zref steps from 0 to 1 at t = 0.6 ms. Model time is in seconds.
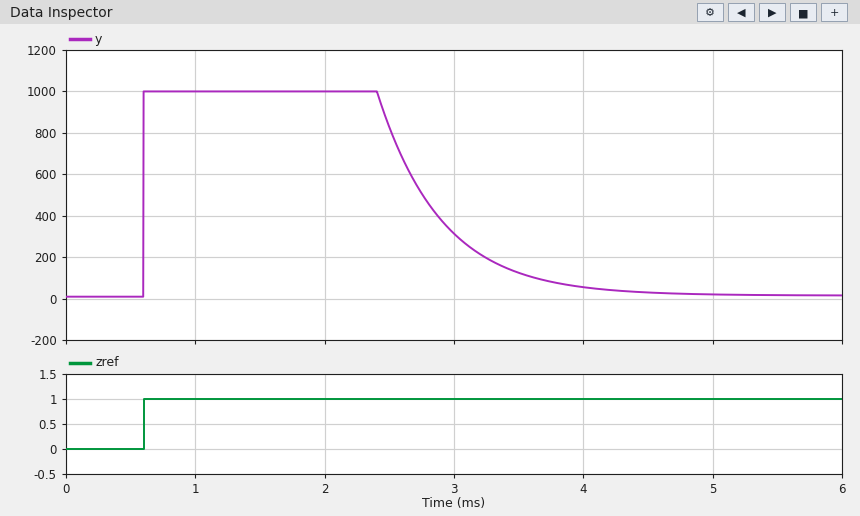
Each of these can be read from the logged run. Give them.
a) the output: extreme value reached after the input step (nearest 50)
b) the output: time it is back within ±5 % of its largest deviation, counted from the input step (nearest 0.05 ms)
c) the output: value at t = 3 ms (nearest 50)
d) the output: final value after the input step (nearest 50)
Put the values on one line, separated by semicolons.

1000; 3.30 ms; 300; 0
